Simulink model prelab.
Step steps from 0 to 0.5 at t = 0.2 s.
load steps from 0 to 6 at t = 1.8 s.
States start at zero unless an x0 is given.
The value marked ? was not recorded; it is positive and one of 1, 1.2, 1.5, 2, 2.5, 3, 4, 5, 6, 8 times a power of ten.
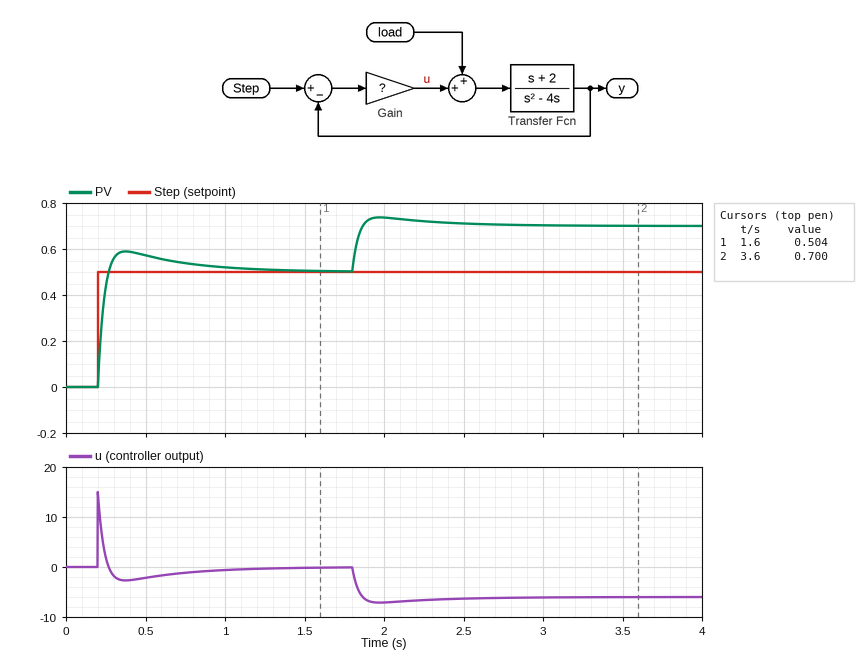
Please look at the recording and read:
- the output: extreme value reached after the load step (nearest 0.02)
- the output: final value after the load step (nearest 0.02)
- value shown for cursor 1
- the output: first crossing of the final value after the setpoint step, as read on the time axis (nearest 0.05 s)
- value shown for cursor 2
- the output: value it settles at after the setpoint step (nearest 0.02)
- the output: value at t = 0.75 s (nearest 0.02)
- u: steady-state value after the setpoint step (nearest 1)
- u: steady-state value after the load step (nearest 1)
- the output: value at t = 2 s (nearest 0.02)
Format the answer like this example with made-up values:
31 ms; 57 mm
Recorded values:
0.74; 0.70; 0.504; 0.25 s; 0.700; 0.50; 0.54; 0; -6; 0.74
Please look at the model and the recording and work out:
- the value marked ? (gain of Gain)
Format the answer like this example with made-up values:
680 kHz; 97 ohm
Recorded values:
30
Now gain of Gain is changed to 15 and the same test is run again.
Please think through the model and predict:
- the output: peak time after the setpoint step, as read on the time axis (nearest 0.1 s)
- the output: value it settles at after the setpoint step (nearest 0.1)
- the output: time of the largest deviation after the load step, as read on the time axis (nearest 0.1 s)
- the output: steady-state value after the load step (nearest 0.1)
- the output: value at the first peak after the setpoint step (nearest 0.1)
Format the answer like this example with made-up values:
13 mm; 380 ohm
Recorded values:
0.5 s; 0.5; 2.1 s; 0.9; 0.7
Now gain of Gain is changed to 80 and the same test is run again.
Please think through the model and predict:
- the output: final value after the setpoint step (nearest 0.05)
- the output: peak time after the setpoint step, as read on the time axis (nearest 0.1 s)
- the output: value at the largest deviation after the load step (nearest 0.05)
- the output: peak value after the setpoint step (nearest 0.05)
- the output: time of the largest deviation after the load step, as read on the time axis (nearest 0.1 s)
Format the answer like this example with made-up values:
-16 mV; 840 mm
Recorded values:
0.50; 0.3 s; 0.60; 0.55; 1.9 s
